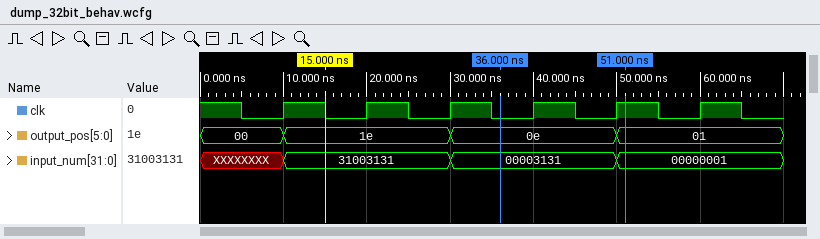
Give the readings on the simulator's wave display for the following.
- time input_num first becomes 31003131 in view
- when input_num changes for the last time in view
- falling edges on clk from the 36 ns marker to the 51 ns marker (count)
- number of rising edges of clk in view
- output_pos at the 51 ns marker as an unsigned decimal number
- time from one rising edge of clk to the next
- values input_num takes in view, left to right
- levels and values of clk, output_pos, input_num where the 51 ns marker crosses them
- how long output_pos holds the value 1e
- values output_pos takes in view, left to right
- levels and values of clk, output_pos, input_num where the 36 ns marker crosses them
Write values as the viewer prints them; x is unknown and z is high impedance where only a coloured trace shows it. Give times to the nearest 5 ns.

10 ns
50 ns
1
6
1
10 ns
XXXXXXXX, 31003131, 00003131, 00000001
clk=1, output_pos=01, input_num=00000001
20 ns
00, 1e, 0e, 01
clk=0, output_pos=0e, input_num=00003131
